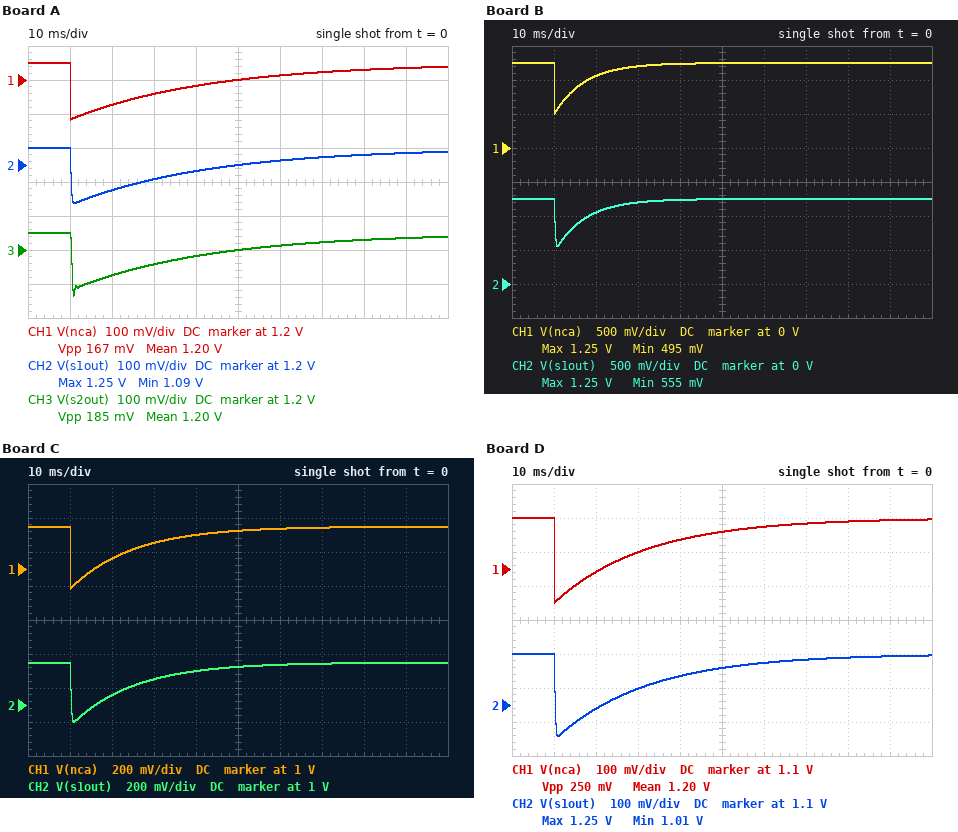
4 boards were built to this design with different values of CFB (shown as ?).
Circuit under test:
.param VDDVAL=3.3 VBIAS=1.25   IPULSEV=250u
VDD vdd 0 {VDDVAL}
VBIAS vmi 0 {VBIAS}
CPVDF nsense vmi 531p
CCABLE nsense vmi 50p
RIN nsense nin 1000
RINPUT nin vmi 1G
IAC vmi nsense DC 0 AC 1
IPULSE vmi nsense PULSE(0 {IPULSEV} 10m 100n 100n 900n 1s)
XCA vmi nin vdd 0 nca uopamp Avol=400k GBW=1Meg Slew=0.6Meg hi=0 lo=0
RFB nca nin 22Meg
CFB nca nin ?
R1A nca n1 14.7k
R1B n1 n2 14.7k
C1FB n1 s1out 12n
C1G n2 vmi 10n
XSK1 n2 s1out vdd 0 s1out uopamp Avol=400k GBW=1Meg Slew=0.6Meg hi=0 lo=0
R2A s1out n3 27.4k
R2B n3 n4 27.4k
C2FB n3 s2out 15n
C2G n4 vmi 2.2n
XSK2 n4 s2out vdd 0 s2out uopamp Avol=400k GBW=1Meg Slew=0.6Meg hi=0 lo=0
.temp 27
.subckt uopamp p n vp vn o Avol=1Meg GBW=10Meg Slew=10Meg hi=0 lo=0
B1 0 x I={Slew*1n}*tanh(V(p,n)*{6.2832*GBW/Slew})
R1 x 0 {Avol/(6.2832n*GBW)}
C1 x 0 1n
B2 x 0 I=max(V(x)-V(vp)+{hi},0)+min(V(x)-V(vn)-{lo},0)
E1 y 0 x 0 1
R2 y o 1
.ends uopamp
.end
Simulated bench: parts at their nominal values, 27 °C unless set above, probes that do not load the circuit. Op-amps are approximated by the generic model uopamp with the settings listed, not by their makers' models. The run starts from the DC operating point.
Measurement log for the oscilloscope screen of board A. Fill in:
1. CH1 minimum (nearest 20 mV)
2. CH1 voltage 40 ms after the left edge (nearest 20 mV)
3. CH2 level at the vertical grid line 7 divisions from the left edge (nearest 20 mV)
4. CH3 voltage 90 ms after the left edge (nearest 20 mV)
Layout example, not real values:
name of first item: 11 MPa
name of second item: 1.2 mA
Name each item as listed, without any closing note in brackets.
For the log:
CH1 minimum: 1.08 V
CH1 voltage 40 ms after the left edge: 1.18 V
CH2 level at the vertical grid line 7 divisions from the left edge: 1.22 V
CH3 voltage 90 ms after the left edge: 1.24 V
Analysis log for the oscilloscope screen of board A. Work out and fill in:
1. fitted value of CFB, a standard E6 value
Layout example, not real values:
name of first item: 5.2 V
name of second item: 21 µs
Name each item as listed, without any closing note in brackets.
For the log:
fitted value of CFB, a standard E6 value: 1.5 nF
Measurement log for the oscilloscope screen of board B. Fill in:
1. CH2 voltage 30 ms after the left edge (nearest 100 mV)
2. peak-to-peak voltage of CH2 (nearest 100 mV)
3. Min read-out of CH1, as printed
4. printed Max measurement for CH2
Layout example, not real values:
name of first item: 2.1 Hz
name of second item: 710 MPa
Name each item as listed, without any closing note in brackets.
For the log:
CH2 voltage 30 ms after the left edge: 1.2 V
peak-to-peak voltage of CH2: 700 mV
Min read-out of CH1, as printed: 495 mV
printed Max measurement for CH2: 1.25 V
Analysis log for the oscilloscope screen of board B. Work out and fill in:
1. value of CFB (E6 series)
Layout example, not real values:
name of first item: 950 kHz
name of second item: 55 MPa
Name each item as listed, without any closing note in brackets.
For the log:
value of CFB: 330 pF
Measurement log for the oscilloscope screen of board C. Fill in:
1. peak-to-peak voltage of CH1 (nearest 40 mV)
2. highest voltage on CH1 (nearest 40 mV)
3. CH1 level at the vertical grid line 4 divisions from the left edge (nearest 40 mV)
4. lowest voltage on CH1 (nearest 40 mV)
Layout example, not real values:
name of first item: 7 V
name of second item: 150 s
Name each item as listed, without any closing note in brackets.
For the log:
peak-to-peak voltage of CH1: 360 mV
highest voltage on CH1: 1.24 V
CH1 level at the vertical grid line 4 divisions from the left edge: 1.20 V
lowest voltage on CH1: 880 mV
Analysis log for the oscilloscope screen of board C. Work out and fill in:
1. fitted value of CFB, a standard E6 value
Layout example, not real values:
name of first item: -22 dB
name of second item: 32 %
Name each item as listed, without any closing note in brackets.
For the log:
fitted value of CFB, a standard E6 value: 680 pF
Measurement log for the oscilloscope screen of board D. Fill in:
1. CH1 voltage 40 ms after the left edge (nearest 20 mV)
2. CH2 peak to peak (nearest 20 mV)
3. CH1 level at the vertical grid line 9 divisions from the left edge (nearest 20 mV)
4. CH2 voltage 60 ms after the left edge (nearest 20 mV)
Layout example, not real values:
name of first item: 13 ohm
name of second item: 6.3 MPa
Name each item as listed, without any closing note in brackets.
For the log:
CH1 voltage 40 ms after the left edge: 1.18 V
CH2 peak to peak: 240 mV
CH1 level at the vertical grid line 9 divisions from the left edge: 1.24 V
CH2 voltage 60 ms after the left edge: 1.22 V
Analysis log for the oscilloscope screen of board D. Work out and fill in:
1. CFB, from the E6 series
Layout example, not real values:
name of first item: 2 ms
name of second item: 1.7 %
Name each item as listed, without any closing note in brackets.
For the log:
CFB, from the E6 series: 1 nF
